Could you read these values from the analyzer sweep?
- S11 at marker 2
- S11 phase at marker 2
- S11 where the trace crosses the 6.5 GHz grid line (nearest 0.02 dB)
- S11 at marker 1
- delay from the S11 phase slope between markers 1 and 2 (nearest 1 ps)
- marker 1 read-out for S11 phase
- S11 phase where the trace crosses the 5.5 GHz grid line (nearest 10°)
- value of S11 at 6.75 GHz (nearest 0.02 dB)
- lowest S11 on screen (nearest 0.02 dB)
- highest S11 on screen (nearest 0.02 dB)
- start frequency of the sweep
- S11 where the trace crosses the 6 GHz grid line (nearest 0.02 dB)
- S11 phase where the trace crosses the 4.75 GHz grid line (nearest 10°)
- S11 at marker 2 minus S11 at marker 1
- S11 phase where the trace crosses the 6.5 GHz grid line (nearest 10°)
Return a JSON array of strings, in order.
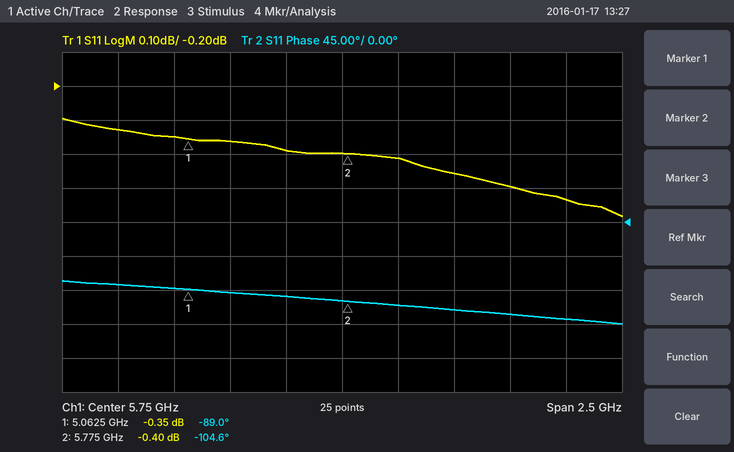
["-0.40 dB", "-104.6°", "-0.50 dB", "-0.35 dB", "61 ps", "-89.0°", "-100°", "-0.54 dB", "-0.58 dB", "-0.30 dB", "4.5 GHz", "-0.42 dB", "-80°", "-0.05 dB", "-120°"]
